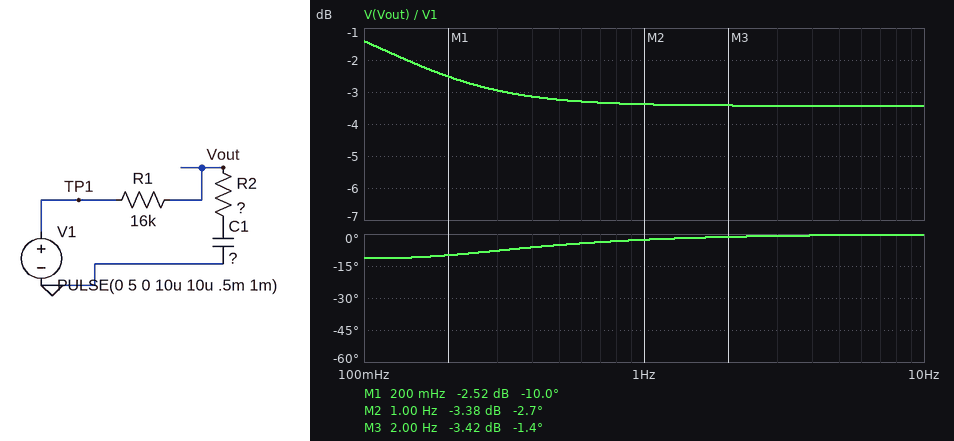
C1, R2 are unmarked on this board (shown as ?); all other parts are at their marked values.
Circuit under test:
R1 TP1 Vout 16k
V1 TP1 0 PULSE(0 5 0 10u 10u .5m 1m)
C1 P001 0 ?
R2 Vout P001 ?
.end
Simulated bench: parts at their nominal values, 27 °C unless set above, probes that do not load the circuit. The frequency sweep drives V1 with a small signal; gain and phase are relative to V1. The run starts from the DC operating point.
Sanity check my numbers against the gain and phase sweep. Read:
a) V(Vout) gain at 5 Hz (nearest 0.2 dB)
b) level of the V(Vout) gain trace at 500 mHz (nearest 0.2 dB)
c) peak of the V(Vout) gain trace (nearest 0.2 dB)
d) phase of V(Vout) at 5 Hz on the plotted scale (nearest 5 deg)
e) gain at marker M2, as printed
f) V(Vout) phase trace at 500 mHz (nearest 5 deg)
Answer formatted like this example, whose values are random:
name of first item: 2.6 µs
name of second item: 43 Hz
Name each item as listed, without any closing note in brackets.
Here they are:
V(Vout) gain at 5 Hz: -3.4 dB
level of the V(Vout) gain trace at 500 mHz: -3.2 dB
peak of the V(Vout) gain trace: -1.4 dB
phase of V(Vout) at 5 Hz on the plotted scale: 0 deg
gain at marker M2, as printed: -3.38 dB
V(Vout) phase trace at 500 mHz: -5 deg
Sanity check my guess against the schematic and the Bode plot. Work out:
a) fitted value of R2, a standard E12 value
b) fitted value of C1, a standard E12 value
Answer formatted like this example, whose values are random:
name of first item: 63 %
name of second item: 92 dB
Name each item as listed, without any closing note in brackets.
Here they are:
fitted value of R2, a standard E12 value: 33 kΩ
fitted value of C1, a standard E12 value: 33 µF
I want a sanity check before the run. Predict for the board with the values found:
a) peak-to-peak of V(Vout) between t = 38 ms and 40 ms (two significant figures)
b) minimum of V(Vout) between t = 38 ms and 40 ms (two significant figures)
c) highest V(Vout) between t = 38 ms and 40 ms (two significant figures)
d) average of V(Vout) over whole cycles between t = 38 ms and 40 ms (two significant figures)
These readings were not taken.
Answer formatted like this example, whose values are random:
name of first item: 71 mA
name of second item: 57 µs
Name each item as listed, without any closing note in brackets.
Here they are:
peak-to-peak of V(Vout) between t = 38 ms and 40 ms: 3.4 V
minimum of V(Vout) between t = 38 ms and 40 ms: 19 mV
highest V(Vout) between t = 38 ms and 40 ms: 3.4 V
average of V(Vout) over whole cycles between t = 38 ms and 40 ms: 1.7 V
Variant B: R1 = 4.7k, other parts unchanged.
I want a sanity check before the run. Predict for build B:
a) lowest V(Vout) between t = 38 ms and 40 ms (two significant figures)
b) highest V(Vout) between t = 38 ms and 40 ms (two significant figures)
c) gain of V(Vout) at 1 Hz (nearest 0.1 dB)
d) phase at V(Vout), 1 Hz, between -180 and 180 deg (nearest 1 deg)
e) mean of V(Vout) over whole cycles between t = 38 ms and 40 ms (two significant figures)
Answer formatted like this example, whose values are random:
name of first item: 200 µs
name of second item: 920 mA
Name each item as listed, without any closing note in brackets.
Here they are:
lowest V(Vout) between t = 38 ms and 40 ms: 9.6 mV
highest V(Vout) between t = 38 ms and 40 ms: 4.4 V
gain of V(Vout) at 1 Hz: -1.1 dB
phase at V(Vout), 1 Hz, between -180 and 180 deg: -1 deg
mean of V(Vout) over whole cycles between t = 38 ms and 40 ms: 2.2 V
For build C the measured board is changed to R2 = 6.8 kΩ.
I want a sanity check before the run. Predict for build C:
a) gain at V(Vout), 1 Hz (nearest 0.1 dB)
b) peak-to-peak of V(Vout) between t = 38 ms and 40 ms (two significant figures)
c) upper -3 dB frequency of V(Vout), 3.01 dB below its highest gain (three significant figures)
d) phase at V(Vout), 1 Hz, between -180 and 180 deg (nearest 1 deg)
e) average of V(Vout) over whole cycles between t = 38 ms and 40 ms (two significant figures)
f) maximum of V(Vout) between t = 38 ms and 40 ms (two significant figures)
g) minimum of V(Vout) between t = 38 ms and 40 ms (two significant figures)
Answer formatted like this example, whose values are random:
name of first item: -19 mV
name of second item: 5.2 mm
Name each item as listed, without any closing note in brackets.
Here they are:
gain at V(Vout), 1 Hz: -8.9 dB
peak-to-peak of V(Vout) between t = 38 ms and 40 ms: 1.5 V
upper -3 dB frequency of V(Vout), 3.01 dB below its highest gain: 233 mHz
phase at V(Vout), 1 Hz, between -180 and 180 deg: -23 deg
average of V(Vout) over whole cycles between t = 38 ms and 40 ms: 850 mV
maximum of V(Vout) between t = 38 ms and 40 ms: 1.6 V
minimum of V(Vout) between t = 38 ms and 40 ms: 88 mV
